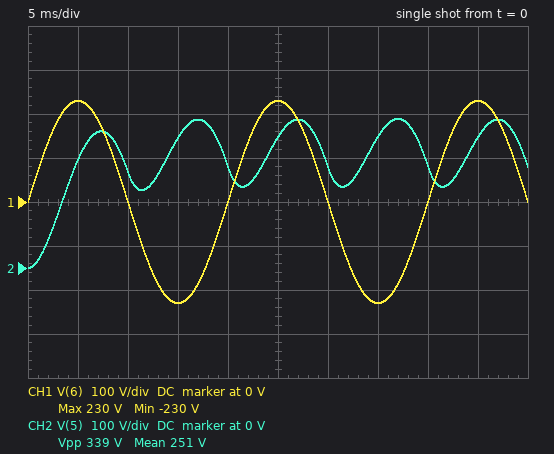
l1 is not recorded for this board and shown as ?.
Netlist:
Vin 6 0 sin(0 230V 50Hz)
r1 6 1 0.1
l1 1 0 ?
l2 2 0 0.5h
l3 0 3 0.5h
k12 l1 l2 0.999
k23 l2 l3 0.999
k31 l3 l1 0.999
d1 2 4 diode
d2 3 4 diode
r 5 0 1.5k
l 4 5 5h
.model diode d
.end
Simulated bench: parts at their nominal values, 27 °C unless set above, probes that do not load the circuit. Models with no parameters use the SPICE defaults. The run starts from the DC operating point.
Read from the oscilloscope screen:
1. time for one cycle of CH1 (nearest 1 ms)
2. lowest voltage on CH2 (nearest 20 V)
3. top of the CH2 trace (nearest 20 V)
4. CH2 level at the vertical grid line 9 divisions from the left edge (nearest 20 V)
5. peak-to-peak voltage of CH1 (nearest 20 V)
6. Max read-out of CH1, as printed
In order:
20 ms
0 V
340 V
300 V
460 V
230 V
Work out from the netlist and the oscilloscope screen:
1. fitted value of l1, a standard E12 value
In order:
150 mH
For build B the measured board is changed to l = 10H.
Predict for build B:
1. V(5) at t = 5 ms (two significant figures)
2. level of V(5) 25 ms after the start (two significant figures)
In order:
150 V
270 V
